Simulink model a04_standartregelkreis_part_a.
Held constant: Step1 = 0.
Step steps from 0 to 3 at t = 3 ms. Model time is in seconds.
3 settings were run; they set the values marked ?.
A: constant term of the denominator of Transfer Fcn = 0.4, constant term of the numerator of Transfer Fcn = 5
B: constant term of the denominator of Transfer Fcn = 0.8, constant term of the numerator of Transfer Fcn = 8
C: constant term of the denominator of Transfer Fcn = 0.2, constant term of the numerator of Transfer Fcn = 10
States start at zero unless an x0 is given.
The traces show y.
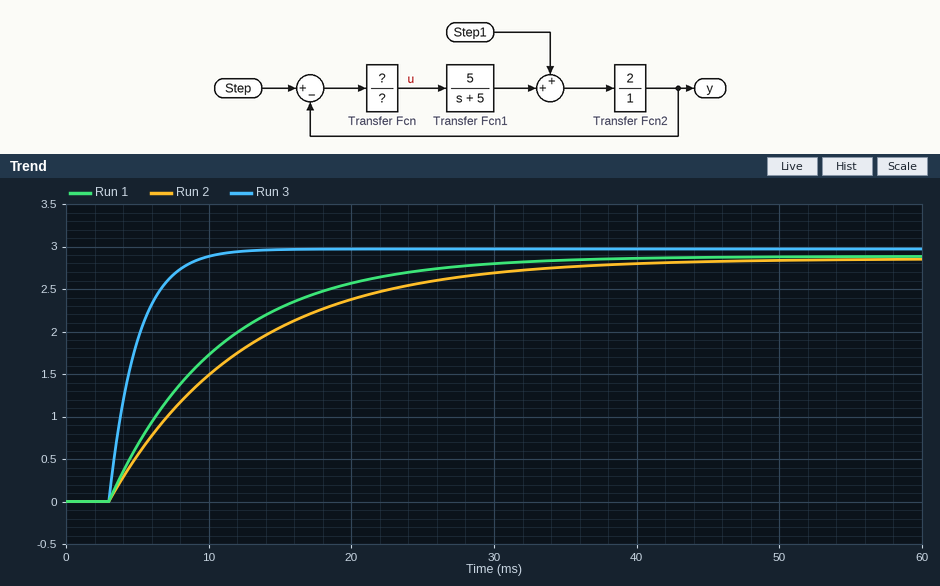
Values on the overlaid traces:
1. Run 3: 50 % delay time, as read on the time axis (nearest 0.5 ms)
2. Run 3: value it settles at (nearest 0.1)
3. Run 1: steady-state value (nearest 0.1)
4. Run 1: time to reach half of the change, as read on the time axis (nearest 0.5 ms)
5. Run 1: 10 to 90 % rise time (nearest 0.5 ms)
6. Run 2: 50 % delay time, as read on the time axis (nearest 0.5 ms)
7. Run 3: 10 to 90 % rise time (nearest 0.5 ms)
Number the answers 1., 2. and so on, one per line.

1. 4.5 ms
2. 3.0
3. 2.9
4. 8.5 ms
5. 17.0 ms
6. 9.5 ms
7. 4.5 ms
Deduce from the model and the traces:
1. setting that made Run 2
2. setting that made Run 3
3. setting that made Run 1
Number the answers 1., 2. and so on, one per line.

1. B
2. C
3. A
